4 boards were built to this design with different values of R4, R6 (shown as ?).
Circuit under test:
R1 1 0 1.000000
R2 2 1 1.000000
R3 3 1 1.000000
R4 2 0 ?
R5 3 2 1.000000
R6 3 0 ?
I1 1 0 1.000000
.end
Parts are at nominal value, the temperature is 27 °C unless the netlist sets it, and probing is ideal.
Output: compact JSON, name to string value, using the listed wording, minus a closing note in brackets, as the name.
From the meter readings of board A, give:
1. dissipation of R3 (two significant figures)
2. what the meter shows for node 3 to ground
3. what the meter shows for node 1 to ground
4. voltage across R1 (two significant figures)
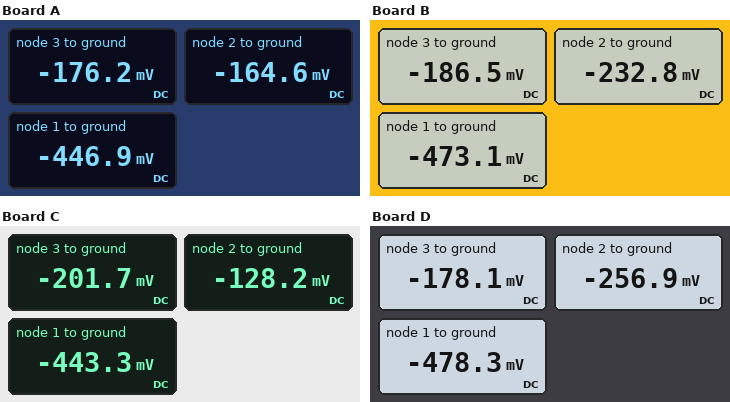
{"dissipation of R3": "73 mW", "what the meter shows for node 3 to ground": "-176.2 mV", "what the meter shows for node 1 to ground": "-446.9 mV", "voltage across R1": "450 mV"}
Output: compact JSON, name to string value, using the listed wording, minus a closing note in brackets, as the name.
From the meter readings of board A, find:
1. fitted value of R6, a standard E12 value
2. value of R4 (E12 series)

{"fitted value of R6, a standard E12 value": "0.68 Ω", "value of R4": "0.56 Ω"}
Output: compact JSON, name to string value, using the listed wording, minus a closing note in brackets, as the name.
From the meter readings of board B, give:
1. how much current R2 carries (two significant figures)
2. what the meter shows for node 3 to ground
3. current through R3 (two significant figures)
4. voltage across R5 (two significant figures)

{"how much current R2 carries": "240 mA", "what the meter shows for node 3 to ground": "-186.5 mV", "current through R3": "290 mA", "voltage across R5": "46 mV"}
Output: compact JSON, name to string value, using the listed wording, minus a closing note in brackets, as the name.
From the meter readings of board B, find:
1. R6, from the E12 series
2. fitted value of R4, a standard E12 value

{"R6, from the E12 series": "0.56 Ω", "fitted value of R4, a standard E12 value": "1.2 Ω"}
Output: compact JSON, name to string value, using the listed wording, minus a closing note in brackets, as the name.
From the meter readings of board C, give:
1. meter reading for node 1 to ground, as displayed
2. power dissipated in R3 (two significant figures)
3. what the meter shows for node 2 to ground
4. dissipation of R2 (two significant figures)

{"meter reading for node 1 to ground, as displayed": "-443.3 mV", "power dissipated in R3": "58 mW", "what the meter shows for node 2 to ground": "-128.2 mV", "dissipation of R2": "99 mW"}
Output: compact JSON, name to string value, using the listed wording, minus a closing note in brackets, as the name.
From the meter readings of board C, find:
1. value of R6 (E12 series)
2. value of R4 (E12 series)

{"value of R6": "1.2 Ω", "value of R4": "0.33 Ω"}
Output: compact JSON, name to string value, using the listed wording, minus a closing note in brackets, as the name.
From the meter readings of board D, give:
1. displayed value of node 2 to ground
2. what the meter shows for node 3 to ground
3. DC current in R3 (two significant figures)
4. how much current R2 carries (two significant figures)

{"displayed value of node 2 to ground": "-256.9 mV", "what the meter shows for node 3 to ground": "-178.1 mV", "DC current in R3": "300 mA", "how much current R2 carries": "220 mA"}
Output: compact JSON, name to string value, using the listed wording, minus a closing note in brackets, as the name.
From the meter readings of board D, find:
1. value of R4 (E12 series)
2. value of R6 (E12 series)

{"value of R4": "1.8 Ω", "value of R6": "0.47 Ω"}
